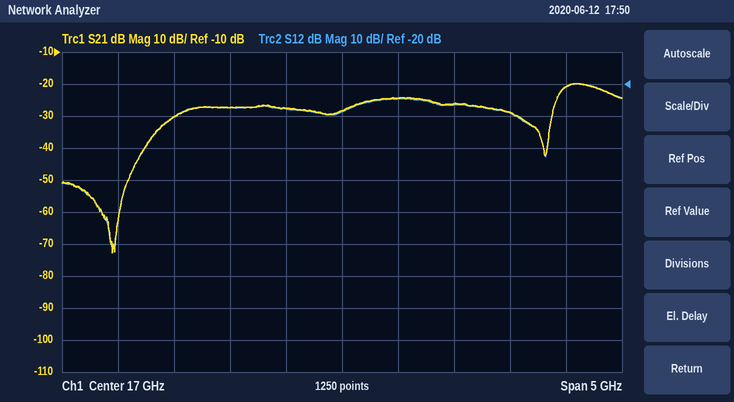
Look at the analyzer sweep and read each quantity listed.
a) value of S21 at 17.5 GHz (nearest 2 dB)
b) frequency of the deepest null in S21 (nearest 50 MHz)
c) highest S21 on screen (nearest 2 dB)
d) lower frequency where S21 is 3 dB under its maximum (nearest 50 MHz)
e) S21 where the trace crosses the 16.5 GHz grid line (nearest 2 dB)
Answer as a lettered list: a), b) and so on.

a) -24 dB
b) 14.95 GHz
c) -20 dB
d) 18.95 GHz
e) -28 dB
